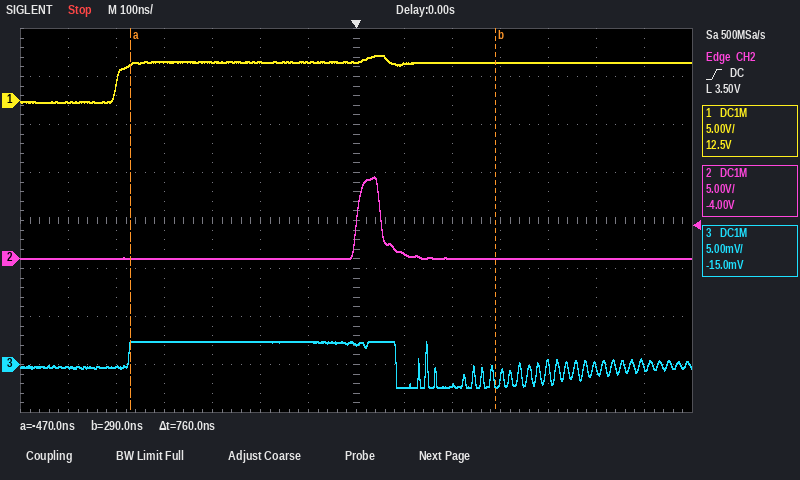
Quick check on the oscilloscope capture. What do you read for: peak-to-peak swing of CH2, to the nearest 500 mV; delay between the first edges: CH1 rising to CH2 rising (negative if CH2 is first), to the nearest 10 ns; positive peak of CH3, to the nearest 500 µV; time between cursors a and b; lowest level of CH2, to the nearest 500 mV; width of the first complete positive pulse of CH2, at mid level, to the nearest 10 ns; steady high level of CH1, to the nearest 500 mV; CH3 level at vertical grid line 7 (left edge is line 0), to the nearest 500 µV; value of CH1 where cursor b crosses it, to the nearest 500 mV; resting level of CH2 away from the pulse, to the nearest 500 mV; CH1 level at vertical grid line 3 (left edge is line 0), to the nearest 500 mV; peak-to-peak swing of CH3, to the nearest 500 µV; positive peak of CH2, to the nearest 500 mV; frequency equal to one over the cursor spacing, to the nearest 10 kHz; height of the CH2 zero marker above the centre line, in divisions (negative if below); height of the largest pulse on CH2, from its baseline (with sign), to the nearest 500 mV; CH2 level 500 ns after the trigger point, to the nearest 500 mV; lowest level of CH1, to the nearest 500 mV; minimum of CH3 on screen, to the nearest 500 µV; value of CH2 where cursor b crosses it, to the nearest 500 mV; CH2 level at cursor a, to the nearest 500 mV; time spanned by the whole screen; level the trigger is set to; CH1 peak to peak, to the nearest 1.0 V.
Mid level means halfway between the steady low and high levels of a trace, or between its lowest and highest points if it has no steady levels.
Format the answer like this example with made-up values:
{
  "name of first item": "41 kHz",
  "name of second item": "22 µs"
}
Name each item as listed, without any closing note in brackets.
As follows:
{
  "peak-to-peak swing of CH2, to the nearest 500 mV": "8.5 V",
  "delay between the first edges: CH1 rising to CH2 rising (negative if CH2 is first), to the nearest 10 ns": "+500 ns",
  "positive peak of CH3, to the nearest 500 µV": "2.5 mV",
  "time between cursors a and b": "760 ns",
  "lowest level of CH2, to the nearest 500 mV": "0.0 V",
  "width of the first complete positive pulse of CH2, at mid level, to the nearest 10 ns": "50 ns",
  "steady high level of CH1, to the nearest 500 mV": "4.0 V",
  "CH3 level at vertical grid line 7 (left edge is line 0), to the nearest 500 µV": "2.0 mV",
  "value of CH1 where cursor b crosses it, to the nearest 500 mV": "4.0 V",
  "resting level of CH2 away from the pulse, to the nearest 500 mV": "0.0 V",
  "CH1 level at vertical grid line 3 (left edge is line 0), to the nearest 500 mV": "4.0 V",
  "peak-to-peak swing of CH3, to the nearest 500 µV": "5.0 mV",
  "positive peak of CH2, to the nearest 500 mV": "8.5 V",
  "frequency equal to one over the cursor spacing, to the nearest 10 kHz": "1.32 MHz",
  "height of the CH2 zero marker above the centre line, in divisions": "-0.8 div",
  "height of the largest pulse on CH2, from its baseline (with sign), to the nearest 500 mV": "+8.5 V",
  "CH2 level 500 ns after the trigger point, to the nearest 500 mV": "0.0 V",
  "lowest level of CH1, to the nearest 500 mV": "0.0 V",
  "minimum of CH3 on screen, to the nearest 500 µV": "-2.5 mV",
  "value of CH2 where cursor b crosses it, to the nearest 500 mV": "0.0 V",
  "CH2 level at cursor a, to the nearest 500 mV": "0.0 V",
  "time spanned by the whole screen": "1.4 µs",
  "level the trigger is set to": "3.50 V",
  "CH1 peak to peak, to the nearest 1.0 V": "5.0 V"
}
